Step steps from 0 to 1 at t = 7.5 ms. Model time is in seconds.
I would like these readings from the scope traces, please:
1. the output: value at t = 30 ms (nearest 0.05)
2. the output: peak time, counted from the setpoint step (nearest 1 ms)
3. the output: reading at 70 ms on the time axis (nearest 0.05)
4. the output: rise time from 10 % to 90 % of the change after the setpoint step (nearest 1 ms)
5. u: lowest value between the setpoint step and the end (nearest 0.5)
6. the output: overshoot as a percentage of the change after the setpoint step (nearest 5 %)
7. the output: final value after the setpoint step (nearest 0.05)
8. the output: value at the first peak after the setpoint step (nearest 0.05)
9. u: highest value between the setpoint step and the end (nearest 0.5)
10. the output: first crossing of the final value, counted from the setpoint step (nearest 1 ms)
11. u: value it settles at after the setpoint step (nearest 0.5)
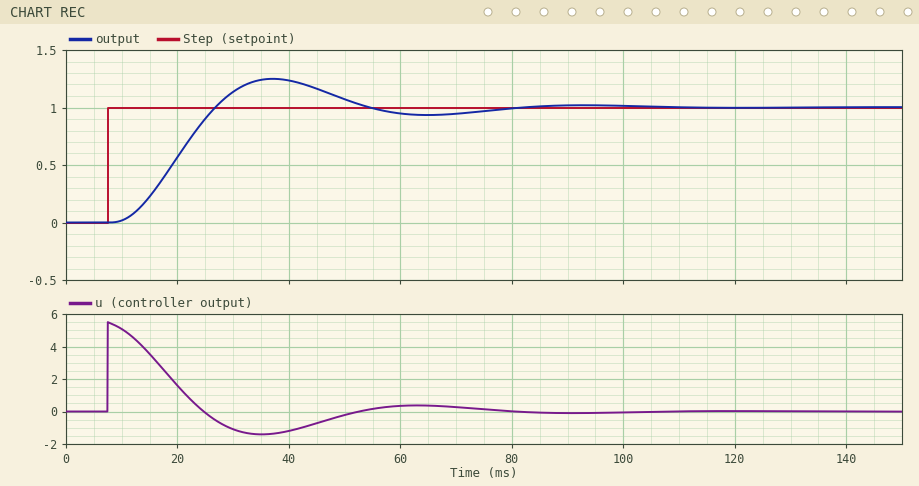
1.15
30 ms
0.95
12 ms
-1.5
25 %
1.00
1.25
5.5
19 ms
0.0
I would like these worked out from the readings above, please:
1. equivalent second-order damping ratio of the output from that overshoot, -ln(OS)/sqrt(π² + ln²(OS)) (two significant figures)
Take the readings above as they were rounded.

0.40
